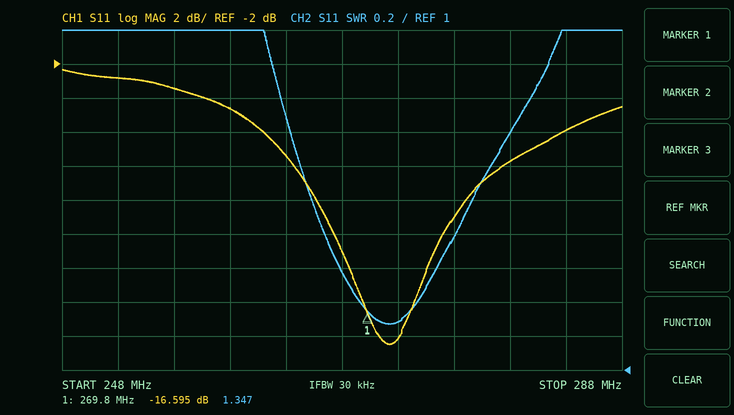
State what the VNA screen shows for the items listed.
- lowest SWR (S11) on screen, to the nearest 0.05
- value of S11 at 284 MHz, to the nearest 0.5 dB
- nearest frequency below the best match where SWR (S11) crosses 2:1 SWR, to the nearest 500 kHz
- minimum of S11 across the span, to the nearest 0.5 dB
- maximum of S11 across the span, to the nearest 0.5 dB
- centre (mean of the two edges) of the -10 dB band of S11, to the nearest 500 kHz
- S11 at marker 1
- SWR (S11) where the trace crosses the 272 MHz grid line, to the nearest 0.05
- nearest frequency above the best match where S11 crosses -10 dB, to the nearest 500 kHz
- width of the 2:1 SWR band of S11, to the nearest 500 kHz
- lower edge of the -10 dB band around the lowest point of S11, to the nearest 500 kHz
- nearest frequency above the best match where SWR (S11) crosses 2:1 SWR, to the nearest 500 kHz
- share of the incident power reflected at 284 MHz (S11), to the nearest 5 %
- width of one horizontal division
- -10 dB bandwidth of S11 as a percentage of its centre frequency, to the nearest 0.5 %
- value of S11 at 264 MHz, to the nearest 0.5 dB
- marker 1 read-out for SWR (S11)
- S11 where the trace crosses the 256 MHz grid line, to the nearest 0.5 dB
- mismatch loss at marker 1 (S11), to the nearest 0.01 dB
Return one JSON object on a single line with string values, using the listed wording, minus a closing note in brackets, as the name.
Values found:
{"lowest SWR (S11) on screen, to the nearest 0.05": "1.25", "value of S11 at 284 MHz, to the nearest 0.5 dB": "-6.0 dB", "nearest frequency below the best match where SWR (S11) crosses 2:1 SWR, to the nearest 500 kHz": "266.0 MHz", "minimum of S11 across the span, to the nearest 0.5 dB": "-18.5 dB", "maximum of S11 across the span, to the nearest 0.5 dB": "-2.5 dB", "centre (mean of the two edges) of the -10 dB band of S11, to the nearest 500 kHz": "271.5 MHz", "S11 at marker 1": "-16.595 dB", "SWR (S11) where the trace crosses the 272 MHz grid line, to the nearest 0.05": "1.30", "nearest frequency above the best match where S11 crosses -10 dB, to the nearest 500 kHz": "277.0 MHz", "width of the 2:1 SWR band of S11, to the nearest 500 kHz": "11.5 MHz", "lower edge of the -10 dB band around the lowest point of S11, to the nearest 500 kHz": "266.0 MHz", "nearest frequency above the best match where SWR (S11) crosses 2:1 SWR, to the nearest 500 kHz": "277.5 MHz", "share of the incident power reflected at 284 MHz (S11), to the nearest 5 %": "25 %", "width of one horizontal division": "4 MHz", "-10 dB bandwidth of S11 as a percentage of its centre frequency, to the nearest 0.5 %": "4.0 %", "value of S11 at 264 MHz, to the nearest 0.5 dB": "-7.5 dB", "marker 1 read-out for SWR": "1.347", "S11 where the trace crosses the 256 MHz grid line, to the nearest 0.5 dB": "-3.5 dB", "mismatch loss at marker 1 (S11), to the nearest 0.01 dB": "0.10 dB"}
